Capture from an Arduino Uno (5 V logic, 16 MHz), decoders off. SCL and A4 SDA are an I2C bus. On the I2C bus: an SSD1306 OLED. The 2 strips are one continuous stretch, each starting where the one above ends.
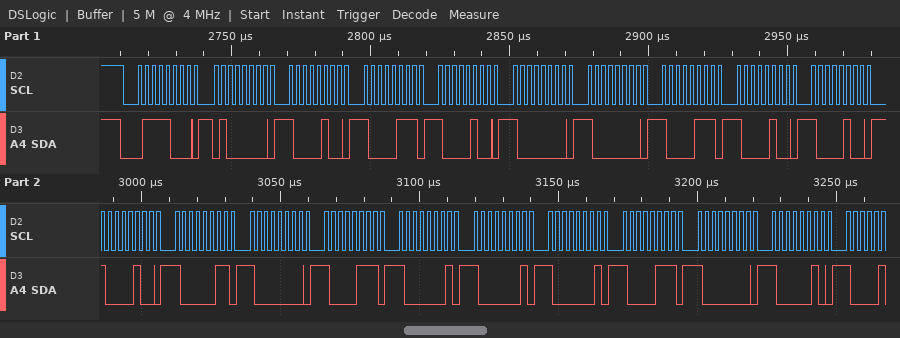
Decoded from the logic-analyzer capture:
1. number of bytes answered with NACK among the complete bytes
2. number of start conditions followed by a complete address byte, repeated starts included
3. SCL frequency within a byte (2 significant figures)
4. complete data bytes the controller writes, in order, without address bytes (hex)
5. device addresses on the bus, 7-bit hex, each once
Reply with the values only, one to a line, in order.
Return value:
0
1
400 kHz
40 84 87 84 80 80 87 84 84 84 83 80 87 81 81 81 87 80 82
0x3C
